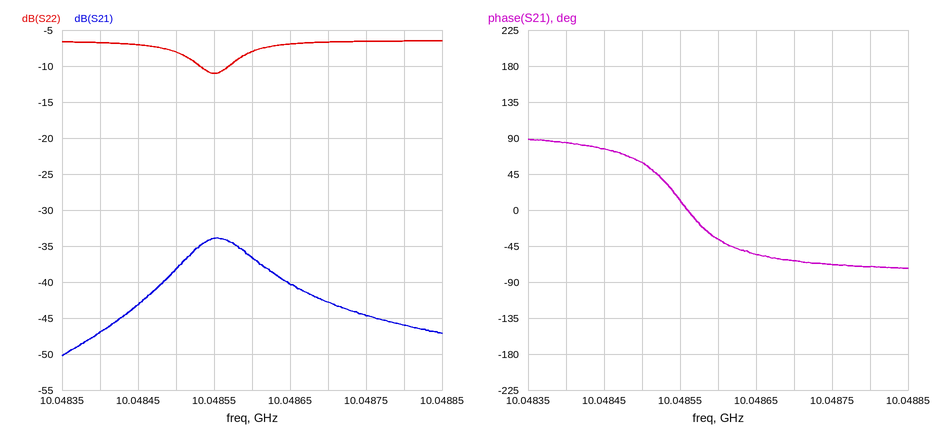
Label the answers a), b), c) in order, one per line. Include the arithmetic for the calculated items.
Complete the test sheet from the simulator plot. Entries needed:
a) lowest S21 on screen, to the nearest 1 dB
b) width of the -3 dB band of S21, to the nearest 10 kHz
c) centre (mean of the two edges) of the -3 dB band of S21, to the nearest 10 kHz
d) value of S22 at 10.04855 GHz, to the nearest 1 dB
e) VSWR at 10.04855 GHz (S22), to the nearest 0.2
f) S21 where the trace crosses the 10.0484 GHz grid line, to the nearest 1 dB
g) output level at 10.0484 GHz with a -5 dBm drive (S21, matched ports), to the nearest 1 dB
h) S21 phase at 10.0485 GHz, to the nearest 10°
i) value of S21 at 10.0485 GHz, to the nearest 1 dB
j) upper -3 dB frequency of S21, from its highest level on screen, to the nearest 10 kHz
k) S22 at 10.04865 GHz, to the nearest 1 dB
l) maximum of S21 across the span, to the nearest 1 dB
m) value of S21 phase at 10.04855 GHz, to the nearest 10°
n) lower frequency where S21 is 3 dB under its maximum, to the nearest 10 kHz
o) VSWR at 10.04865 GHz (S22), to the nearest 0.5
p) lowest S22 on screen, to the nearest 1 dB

a) -50 dB
b) 10.04860 GHz − 10.04851 GHz = 90 kHz
c) 10.04856 GHz
d) -11 dB
e) |Γ| = 10^(-11/20) = 0.2818; VSWR = (1 + 0.2818)/(1 − 0.2818) ≈ 1.8
f) -47 dB
g) -5 dBm + (-47 dB) = -52 dBm
h) 60°
i) -38 dB
j) 10.04860 GHz
k) -7 dB
l) -34 dB
m) 10°
n) 10.04851 GHz
o) |Γ| = 10^(-7/20) = 0.4467; VSWR = (1 + 0.4467)/(1 − 0.4467) ≈ 2.61, so 2.5 to the nearest 0.5
p) -11 dB
